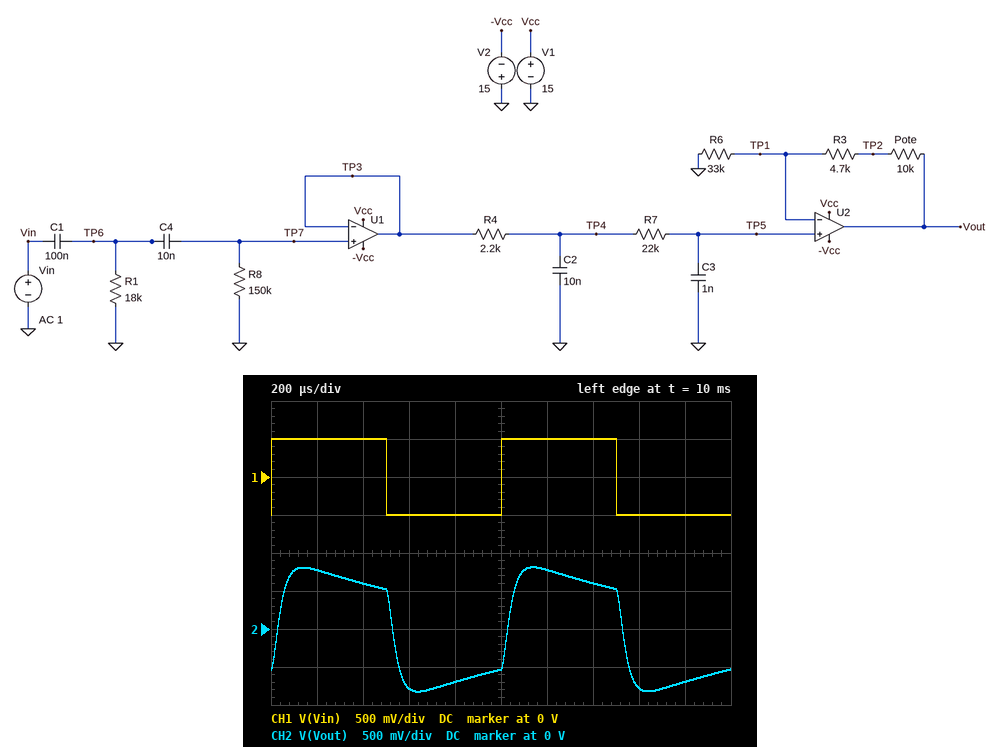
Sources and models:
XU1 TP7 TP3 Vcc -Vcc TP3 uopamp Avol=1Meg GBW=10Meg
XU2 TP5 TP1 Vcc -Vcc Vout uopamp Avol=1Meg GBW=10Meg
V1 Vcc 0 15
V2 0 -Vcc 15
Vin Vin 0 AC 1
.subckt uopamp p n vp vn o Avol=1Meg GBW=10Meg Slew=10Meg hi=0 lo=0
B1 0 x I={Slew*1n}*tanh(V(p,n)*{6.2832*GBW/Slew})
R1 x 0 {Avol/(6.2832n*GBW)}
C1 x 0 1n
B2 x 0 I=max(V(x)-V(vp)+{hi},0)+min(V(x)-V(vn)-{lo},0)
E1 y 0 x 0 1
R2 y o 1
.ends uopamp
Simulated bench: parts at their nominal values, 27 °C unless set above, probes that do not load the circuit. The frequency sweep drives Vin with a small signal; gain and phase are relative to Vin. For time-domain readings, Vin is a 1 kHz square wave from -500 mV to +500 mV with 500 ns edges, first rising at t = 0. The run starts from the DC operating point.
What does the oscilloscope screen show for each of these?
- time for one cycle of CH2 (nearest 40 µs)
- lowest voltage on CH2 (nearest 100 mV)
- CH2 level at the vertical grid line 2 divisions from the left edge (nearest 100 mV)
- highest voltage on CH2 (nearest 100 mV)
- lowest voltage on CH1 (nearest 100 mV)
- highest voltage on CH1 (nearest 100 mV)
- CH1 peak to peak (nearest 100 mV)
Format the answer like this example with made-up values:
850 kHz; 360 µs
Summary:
1.00 ms; -800 mV; 600 mV; 800 mV; -500 mV; 500 mV; 1.0 V
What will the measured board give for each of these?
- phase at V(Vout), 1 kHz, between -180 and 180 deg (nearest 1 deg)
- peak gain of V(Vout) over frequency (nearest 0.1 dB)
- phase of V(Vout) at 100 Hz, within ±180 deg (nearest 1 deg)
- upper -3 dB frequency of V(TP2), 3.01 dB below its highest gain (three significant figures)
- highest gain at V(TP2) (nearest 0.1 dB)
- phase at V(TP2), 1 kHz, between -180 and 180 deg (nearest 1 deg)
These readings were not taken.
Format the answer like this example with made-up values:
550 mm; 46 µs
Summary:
-5 deg; 2.9 dB; 87 deg; 4.59 kHz; 0.9 dB; -5 deg
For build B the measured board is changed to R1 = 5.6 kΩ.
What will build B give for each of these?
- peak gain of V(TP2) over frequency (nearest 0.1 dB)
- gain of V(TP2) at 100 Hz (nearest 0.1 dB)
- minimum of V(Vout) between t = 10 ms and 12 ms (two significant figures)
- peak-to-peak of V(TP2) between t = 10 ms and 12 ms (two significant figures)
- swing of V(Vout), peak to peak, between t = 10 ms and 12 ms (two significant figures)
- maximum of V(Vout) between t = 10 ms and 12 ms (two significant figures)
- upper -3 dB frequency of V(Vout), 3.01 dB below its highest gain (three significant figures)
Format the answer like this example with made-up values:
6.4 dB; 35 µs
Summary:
0.6 dB; -11.9 dB; -900 mV; 1.4 V; 1.8 V; 900 mV; 4.83 kHz
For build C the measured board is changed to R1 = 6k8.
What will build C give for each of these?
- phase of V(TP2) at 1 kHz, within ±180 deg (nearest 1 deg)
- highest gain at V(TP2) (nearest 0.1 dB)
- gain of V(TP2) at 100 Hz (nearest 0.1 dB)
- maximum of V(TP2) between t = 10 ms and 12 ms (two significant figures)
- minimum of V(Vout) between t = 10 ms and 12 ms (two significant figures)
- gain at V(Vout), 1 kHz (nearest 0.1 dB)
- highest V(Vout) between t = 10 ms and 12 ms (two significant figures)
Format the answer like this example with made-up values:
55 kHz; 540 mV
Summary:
3 deg; 0.7 dB; -10.5 dB; 700 mV; -880 mV; 2.7 dB; 880 mV
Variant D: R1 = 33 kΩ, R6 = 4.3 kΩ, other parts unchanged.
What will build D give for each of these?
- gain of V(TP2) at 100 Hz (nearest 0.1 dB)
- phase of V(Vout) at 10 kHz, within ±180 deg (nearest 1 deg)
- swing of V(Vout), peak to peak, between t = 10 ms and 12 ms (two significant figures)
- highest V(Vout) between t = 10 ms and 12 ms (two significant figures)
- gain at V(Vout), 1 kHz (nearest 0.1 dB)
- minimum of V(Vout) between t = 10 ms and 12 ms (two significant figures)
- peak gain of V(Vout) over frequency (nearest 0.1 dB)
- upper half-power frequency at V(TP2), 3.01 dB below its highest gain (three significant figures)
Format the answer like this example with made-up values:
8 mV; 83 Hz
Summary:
1.7 dB; -107 deg; 4.9 V; 2.4 V; 12.6 dB; -2.5 V; 12.7 dB; 4.55 kHz
